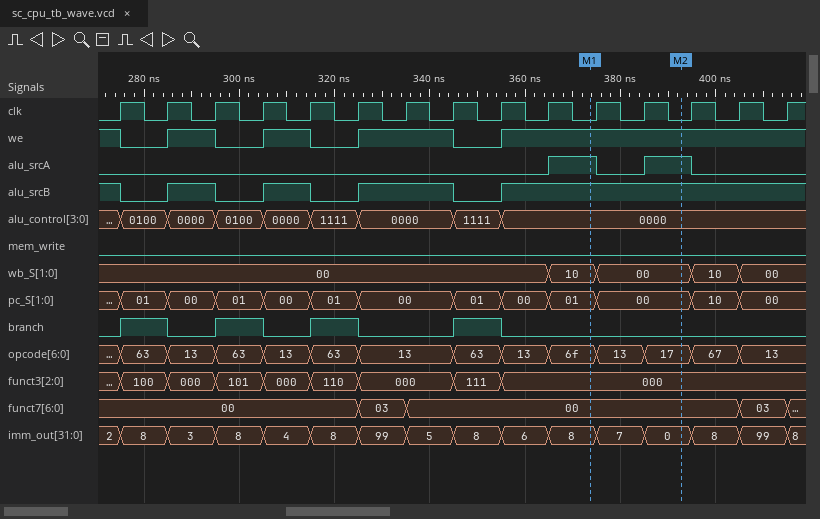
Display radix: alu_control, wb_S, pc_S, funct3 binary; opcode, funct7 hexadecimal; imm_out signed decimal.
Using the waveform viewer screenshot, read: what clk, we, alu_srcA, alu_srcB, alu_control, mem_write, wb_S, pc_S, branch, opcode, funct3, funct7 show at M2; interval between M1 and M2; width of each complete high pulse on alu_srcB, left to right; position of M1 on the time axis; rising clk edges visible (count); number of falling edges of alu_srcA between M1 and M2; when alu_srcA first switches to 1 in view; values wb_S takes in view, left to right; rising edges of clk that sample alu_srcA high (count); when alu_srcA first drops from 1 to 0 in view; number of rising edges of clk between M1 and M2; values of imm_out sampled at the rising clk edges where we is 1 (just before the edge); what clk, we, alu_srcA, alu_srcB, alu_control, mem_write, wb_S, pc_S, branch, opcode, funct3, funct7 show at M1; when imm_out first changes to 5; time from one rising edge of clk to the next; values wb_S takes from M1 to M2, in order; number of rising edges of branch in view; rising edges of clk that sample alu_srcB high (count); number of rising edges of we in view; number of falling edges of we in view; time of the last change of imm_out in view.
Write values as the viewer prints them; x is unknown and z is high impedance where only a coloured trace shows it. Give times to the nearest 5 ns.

clk=0, we=1, alu_srcA=1, alu_srcB=1, alu_control=0000, mem_write=0, wb_S=00, pc_S=00, branch=0, opcode=17, funct3=000, funct7=00
20 ns
10 ns, 10 ns, 20 ns
375 ns
15
1
365 ns
00, 10, 00, 10, 00
2
375 ns
2
2, 3, 4, 99, 5, 6, 8, 7, 0, 8, 99
clk=0, we=1, alu_srcA=1, alu_srcB=1, alu_control=0000, mem_write=0, wb_S=10, pc_S=01, branch=0, opcode=6f, funct3=000, funct7=00
335 ns
10 ns
10, 00
4
11
4
4
415 ns
